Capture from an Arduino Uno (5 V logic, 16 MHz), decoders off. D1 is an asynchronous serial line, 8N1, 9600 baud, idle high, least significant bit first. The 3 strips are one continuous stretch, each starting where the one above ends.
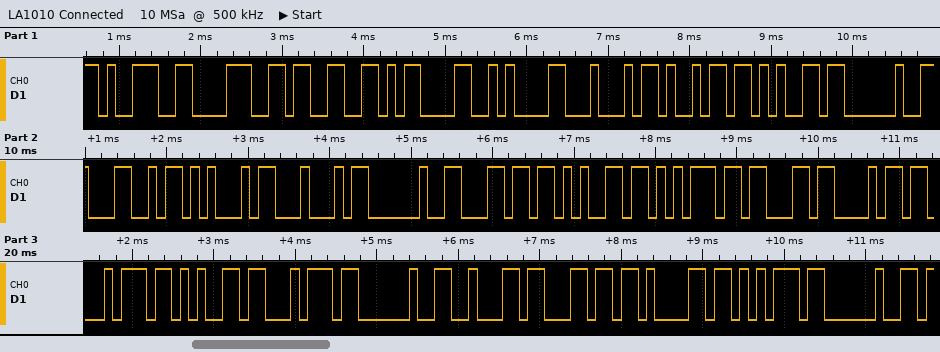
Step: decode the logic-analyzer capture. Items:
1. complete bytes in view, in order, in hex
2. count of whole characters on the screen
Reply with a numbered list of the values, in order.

1. 39 38 33 0D 0A 44 69 65 20 4C 45 44 20 6C 65 75 63 68 74 65 74 20 62 6C 61 75 20
2. 27
